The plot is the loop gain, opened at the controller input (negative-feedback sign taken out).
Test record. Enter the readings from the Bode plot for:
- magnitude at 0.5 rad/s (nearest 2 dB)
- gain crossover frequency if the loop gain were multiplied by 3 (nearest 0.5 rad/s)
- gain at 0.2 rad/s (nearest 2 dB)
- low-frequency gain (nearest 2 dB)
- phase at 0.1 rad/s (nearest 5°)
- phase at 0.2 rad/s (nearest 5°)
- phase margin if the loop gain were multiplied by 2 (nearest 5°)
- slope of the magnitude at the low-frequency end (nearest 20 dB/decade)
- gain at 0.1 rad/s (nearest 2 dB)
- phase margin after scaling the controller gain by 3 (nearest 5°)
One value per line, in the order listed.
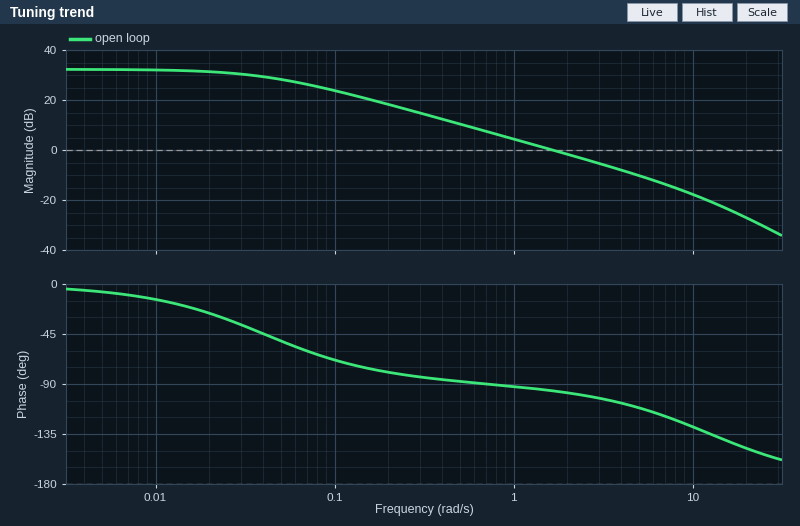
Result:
10 dB
4.5 rad/s
18 dB
32 dB
-70°
-80°
75°
0 dB/decade
24 dB
70°
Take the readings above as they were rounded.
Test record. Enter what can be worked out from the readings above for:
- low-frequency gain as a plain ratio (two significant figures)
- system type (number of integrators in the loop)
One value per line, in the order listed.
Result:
40
0
